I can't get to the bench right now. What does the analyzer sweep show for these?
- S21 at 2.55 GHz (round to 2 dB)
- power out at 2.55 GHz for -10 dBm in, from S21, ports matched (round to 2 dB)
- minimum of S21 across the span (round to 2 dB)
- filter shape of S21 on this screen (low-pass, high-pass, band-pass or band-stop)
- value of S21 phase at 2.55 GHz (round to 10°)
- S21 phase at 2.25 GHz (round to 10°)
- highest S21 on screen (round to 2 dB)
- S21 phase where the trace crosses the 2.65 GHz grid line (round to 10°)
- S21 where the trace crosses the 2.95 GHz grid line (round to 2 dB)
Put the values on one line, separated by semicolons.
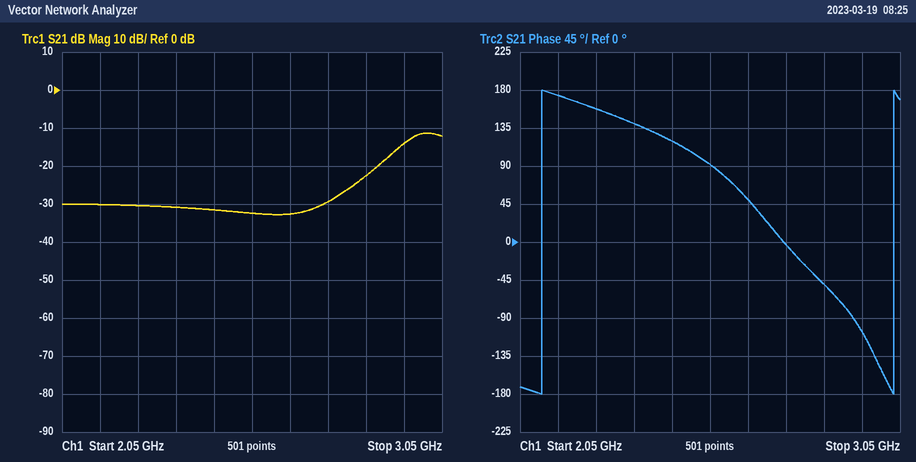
-32 dB; -42 dBm; -32 dB; high-pass; 90°; 160°; -12 dB; 50°; -14 dB
